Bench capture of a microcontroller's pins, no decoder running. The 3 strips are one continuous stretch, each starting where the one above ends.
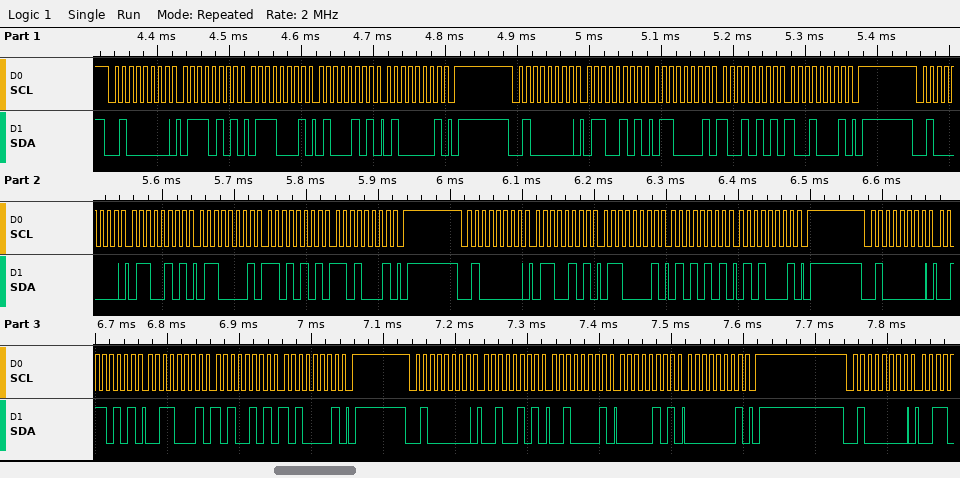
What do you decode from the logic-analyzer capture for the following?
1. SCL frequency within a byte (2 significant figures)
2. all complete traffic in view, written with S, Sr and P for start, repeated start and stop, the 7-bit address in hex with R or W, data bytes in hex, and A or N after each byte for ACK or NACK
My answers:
100 kHz
S 20W A 75 A 71 A 45 A 41 A P S 20W A 65 A 61 A 95 A 91 A P S 20W A 65 A 61 A D5 A D1 A P S 20W A 65 A 61 A 55 A 51 A P S 20W A 35 A 31 A A5 A A1 A P S 20W A 25 A 21 A 05 A 01 A P S 20W A
